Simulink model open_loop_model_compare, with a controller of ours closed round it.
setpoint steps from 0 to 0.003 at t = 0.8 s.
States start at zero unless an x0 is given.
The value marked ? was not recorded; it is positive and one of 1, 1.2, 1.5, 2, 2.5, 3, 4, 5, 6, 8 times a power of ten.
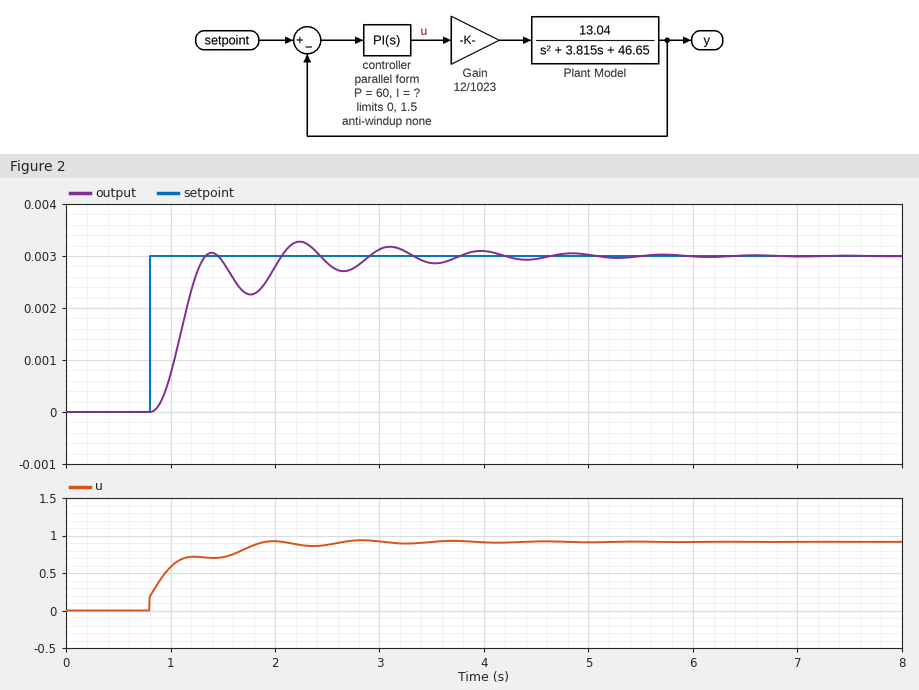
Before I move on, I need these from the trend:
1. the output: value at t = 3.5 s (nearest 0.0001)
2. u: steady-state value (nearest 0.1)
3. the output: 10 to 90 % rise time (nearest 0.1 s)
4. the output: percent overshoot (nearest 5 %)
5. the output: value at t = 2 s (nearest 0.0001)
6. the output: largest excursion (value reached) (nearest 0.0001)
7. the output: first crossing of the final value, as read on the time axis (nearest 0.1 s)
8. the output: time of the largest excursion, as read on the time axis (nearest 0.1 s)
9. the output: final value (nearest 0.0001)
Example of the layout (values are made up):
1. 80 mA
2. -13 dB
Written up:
1. 0.0029
2. 0.9
3. 0.3 s
4. 10 %
5. 0.0028
6. 0.0033
7. 1.3 s
8. 2.2 s
9. 0.0030
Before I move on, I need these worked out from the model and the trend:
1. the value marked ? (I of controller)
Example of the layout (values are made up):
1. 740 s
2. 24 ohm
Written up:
1. 800
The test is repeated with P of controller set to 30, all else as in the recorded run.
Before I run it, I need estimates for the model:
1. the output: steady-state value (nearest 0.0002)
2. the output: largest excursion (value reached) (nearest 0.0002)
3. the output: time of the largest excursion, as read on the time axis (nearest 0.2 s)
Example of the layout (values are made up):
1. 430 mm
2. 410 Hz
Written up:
1. 0.0030
2. 0.0034
3. 2.4 s
